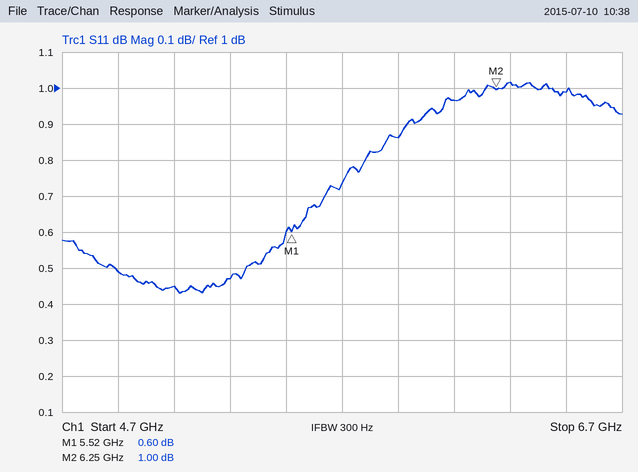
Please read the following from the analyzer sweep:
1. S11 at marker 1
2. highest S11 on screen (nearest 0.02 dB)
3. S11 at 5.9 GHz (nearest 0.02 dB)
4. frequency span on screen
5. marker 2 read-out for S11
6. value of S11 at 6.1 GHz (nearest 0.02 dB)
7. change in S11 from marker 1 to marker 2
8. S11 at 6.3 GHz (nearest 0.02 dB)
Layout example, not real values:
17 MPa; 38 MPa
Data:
0.60 dB; 1.02 dB; 0.86 dB; 2 GHz; 1.00 dB; 0.96 dB; 0.40 dB; 1.02 dB
